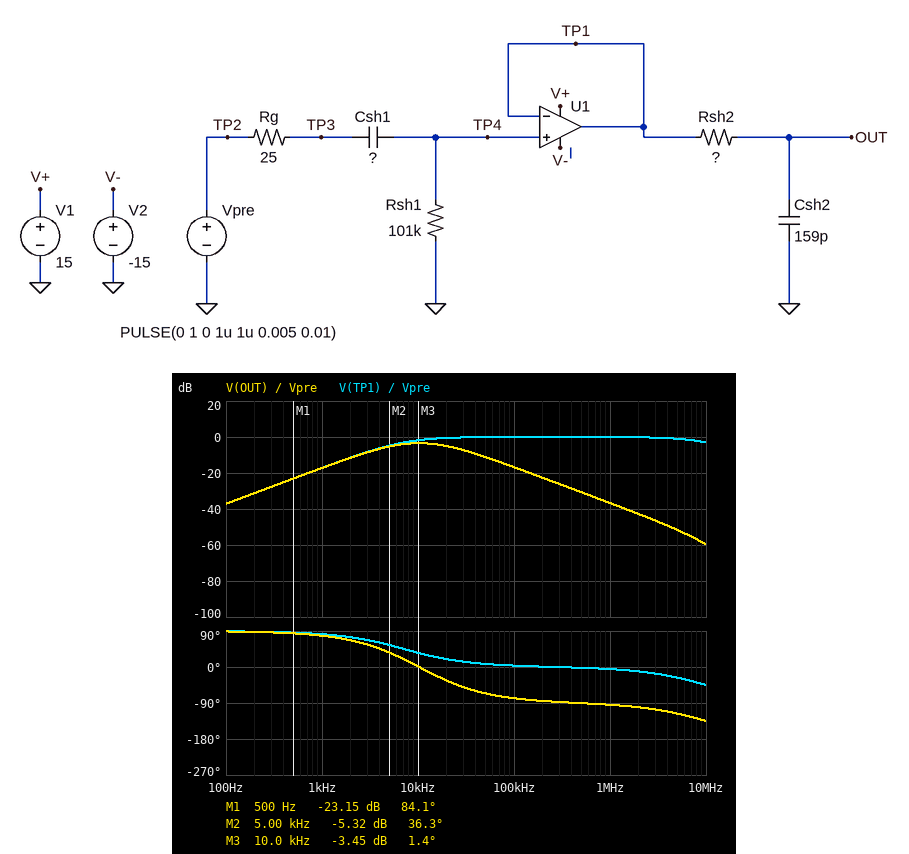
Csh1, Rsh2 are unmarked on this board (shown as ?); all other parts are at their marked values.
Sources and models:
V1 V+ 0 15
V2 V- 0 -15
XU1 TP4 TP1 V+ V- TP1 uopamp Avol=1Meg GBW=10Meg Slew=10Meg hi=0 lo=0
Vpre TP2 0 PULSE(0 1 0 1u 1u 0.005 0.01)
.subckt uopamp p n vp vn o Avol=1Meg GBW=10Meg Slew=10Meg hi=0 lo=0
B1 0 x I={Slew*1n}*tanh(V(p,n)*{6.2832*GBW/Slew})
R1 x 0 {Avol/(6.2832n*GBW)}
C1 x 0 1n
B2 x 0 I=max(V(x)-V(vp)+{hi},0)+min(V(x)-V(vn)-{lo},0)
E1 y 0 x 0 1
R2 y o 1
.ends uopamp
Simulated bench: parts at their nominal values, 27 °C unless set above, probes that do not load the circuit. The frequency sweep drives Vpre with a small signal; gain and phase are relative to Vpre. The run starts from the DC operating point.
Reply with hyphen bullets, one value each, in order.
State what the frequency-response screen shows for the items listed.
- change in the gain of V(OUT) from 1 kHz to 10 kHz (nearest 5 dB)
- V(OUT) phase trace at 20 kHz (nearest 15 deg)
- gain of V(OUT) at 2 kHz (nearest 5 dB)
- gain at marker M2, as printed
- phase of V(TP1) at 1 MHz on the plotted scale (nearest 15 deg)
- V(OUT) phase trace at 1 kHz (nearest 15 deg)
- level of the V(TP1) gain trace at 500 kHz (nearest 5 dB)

- 15 dB
- -30 deg
- -10 dB
- -5.32 dB
- 0 deg
- 75 deg
- 0 dB
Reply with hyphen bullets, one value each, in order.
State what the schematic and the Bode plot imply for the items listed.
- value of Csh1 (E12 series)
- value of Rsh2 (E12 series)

- 220 pF
- 68 kΩ
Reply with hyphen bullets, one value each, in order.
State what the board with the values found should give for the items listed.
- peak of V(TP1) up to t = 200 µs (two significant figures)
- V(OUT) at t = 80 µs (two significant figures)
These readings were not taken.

- 980 mV
- 53 mV
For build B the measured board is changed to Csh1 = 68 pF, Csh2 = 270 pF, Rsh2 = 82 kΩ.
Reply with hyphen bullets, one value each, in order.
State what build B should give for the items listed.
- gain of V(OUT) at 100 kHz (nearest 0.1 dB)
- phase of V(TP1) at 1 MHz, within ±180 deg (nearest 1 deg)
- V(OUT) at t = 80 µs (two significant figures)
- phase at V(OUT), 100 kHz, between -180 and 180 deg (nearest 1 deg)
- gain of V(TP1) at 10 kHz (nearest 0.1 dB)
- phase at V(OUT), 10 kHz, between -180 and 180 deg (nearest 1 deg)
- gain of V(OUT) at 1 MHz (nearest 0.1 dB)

- -23.1 dB
- -4 deg
- 12 mV
- -73 deg
- -8.0 dB
- 12 deg
- -42.9 dB
